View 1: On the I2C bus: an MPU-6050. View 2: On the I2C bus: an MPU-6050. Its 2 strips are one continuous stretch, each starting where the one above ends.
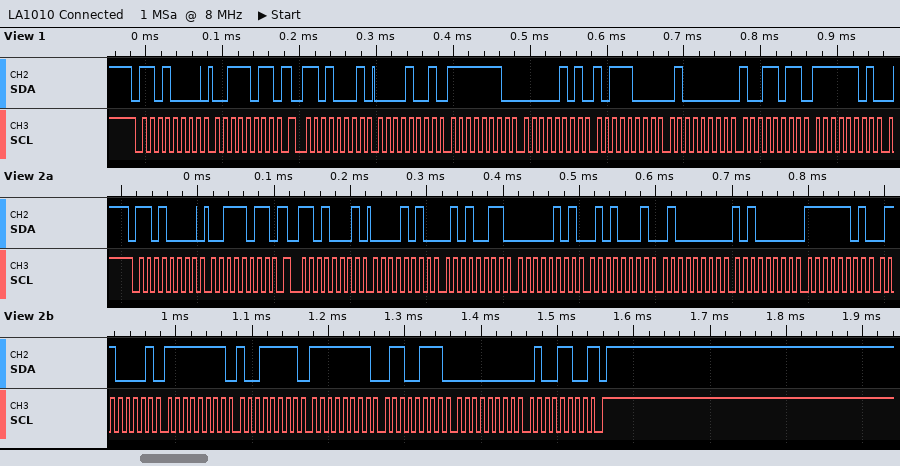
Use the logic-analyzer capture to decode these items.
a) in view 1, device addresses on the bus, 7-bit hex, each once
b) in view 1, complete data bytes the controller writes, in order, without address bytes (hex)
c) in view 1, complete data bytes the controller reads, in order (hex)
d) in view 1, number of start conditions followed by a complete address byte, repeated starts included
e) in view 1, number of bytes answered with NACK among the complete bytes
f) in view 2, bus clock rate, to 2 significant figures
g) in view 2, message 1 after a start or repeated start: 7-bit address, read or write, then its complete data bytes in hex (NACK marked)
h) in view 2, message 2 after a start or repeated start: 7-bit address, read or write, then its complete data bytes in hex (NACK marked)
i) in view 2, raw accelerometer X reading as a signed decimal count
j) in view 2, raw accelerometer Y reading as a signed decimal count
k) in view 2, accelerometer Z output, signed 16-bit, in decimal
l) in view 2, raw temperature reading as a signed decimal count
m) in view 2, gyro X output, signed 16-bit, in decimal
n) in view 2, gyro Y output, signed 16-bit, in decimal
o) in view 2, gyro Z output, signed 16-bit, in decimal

0x68
3B
09 FE 05 B8 40 9B FD
2
0
100 kHz
0x68 write: 3B
0x68 read: 0A 53 05 51 40 A0 FD 61 FF 9F FF 67 00 4C NACK
2643
1361
16544
-671
-97
-153
76
